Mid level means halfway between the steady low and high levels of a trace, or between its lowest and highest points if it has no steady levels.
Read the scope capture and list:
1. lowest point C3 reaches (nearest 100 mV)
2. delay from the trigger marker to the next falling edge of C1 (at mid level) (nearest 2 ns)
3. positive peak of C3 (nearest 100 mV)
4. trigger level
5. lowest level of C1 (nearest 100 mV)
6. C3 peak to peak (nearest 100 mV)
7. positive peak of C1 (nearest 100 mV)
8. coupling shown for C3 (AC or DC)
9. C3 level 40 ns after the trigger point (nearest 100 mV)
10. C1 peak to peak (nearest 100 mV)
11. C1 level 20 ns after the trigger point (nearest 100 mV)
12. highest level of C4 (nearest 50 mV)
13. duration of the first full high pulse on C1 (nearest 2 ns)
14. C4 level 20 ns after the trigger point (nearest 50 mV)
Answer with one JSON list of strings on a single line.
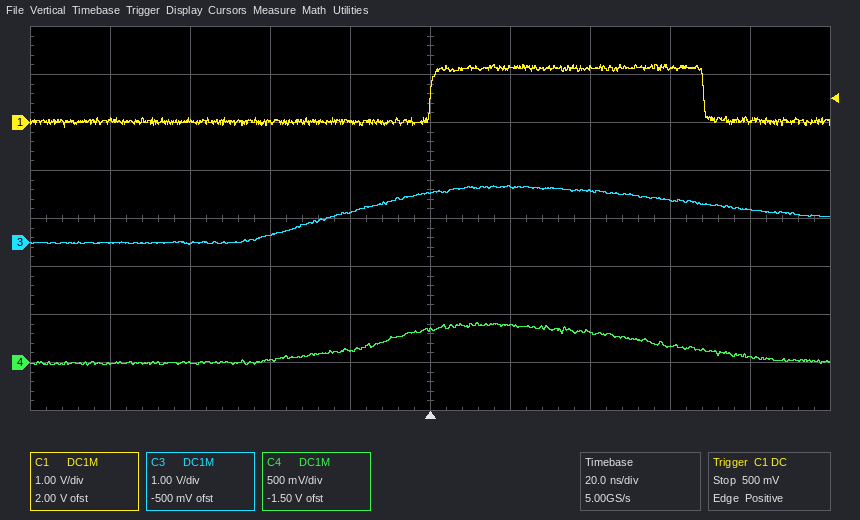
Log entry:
["0.0 V", "68 ns", "1.2 V", "500 mV", "-100 mV", "1.2 V", "1.2 V", "DC", "1.1 V", "1.3 V", "1.1 V", "400 mV", "68 ns", "400 mV"]
